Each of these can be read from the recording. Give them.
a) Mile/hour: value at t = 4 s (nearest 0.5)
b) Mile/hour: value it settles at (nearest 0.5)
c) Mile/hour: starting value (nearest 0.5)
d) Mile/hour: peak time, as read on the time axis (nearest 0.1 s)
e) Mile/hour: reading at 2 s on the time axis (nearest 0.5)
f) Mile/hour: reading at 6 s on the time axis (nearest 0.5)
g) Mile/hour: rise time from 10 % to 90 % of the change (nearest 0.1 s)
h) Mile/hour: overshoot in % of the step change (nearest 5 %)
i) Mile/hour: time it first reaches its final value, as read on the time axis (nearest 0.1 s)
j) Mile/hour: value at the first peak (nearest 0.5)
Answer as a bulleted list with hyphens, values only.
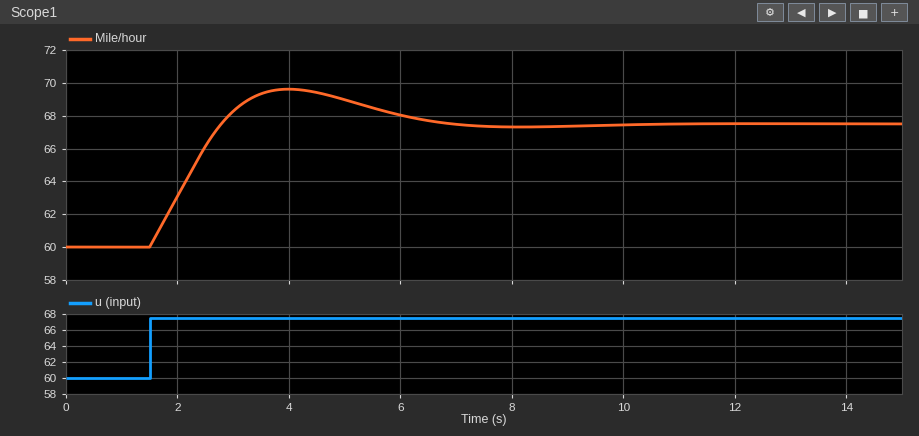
- 69.5
- 67.5
- 60.0
- 4.0 s
- 63.0
- 68.0
- 1.0 s
- 30 %
- 2.8 s
- 69.5
